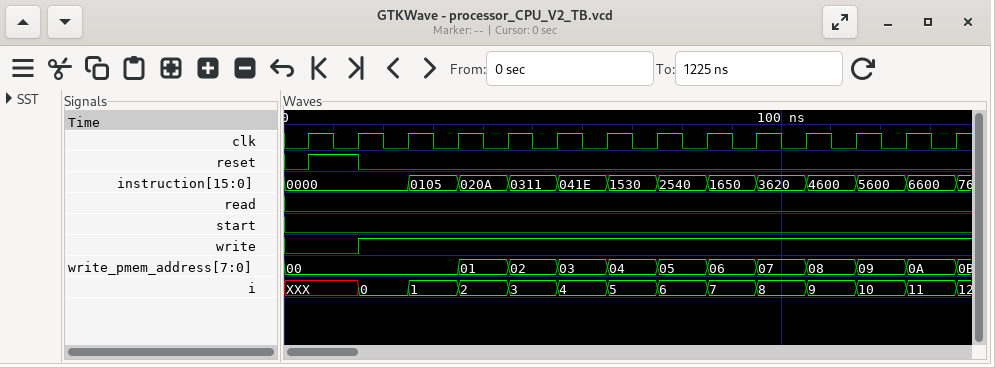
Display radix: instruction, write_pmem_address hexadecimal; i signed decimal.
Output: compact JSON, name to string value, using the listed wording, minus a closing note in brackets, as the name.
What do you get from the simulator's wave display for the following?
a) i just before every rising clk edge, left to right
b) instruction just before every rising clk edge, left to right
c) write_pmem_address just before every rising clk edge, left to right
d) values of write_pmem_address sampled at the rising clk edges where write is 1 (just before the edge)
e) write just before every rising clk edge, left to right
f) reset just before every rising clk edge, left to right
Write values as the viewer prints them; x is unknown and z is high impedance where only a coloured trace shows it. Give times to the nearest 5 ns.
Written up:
{"i just before every rising clk edge, left to right": "XXX, XXX, 0, 1, 2, 3, 4, 5, 6, 7, 8, 9, 10, 11", "instruction just before every rising clk edge, left to right": "0000, 0000, 0000, 0105, 020A, 0311, 041E, 1530, 2540, 1650, 3620, 4600, 5600, 6600", "write_pmem_address just before every rising clk edge, left to right": "00, 00, 00, 00, 01, 02, 03, 04, 05, 06, 07, 08, 09, 0A", "values of write_pmem_address sampled at the rising clk edges where write is 1": "00, 00, 01, 02, 03, 04, 05, 06, 07, 08, 09, 0A", "write just before every rising clk edge, left to right": "0 0 1 1 1 1 1 1 1 1 1 1 1 1", "reset just before every rising clk edge, left to right": "0 1 0 0 0 0 0 0 0 0 0 0 0 0"}
